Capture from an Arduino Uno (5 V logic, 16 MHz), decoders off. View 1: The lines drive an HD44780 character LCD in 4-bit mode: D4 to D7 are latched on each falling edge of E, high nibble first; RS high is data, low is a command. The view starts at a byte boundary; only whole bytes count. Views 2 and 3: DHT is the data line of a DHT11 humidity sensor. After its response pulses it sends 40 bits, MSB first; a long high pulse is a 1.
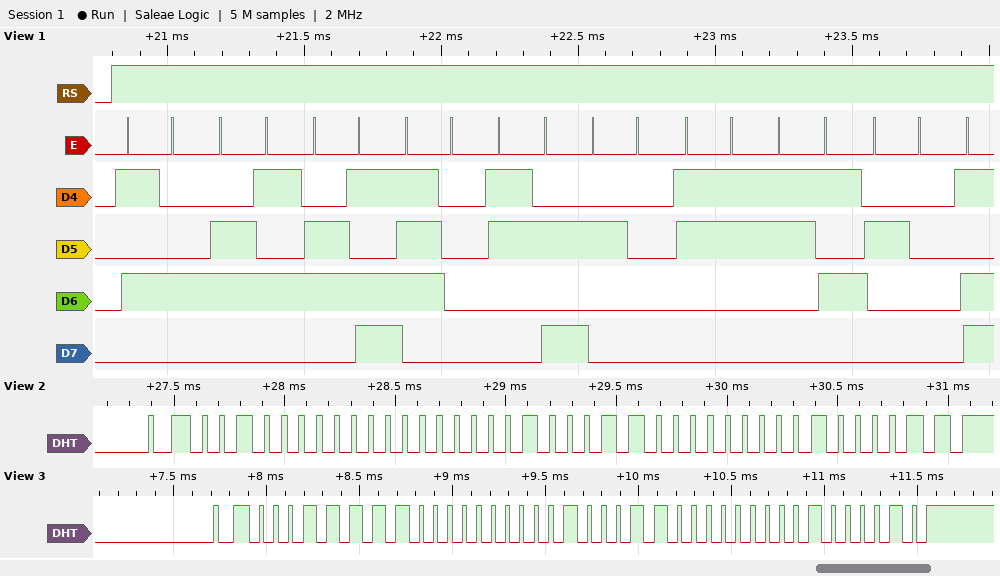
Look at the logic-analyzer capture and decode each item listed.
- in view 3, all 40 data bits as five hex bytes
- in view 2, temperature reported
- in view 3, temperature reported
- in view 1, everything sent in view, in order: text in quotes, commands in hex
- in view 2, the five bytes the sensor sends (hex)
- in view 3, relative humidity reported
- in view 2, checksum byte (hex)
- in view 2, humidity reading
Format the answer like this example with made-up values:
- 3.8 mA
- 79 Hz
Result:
- 1F 00 23 00 42
- 35.0 °C
- 35.0 °C
- "Temp: 35 "
- 20 00 23 00 43
- 31 %
- 0x43
- 32 %
